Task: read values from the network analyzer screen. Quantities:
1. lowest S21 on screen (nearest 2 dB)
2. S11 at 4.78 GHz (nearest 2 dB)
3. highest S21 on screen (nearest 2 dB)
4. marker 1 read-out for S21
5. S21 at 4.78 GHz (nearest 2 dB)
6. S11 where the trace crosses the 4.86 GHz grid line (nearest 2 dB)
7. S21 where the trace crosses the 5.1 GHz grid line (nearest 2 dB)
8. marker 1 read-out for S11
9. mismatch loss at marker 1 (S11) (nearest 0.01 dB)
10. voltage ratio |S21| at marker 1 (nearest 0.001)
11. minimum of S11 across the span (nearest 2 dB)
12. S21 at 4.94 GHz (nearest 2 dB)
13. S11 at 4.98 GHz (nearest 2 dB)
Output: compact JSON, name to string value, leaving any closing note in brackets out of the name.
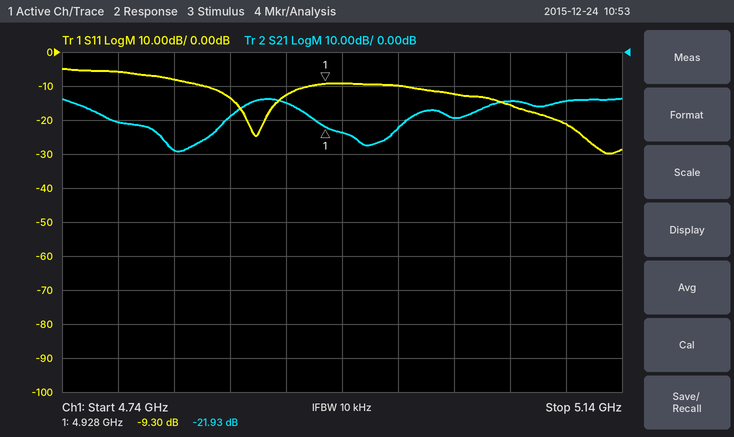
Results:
{"lowest S21 on screen": "-30 dB", "S11 at 4.78 GHz": "-6 dB", "highest S21 on screen": "-14 dB", "marker 1 read-out for S21": "-21.93 dB", "S21 at 4.78 GHz": "-20 dB", "S11 where the trace crosses the 4.86 GHz grid line": "-14 dB", "S21 where the trace crosses the 5.1 GHz grid line": "-14 dB", "marker 1 read-out for S11": "-9.30 dB", "mismatch loss at marker 1 (S11)": "0.54 dB", "voltage ratio |S21| at marker 1": "0.080", "minimum of S11 across the span": "-30 dB", "S21 at 4.94 GHz": "-24 dB", "S11 at 4.98 GHz": "-10 dB"}
